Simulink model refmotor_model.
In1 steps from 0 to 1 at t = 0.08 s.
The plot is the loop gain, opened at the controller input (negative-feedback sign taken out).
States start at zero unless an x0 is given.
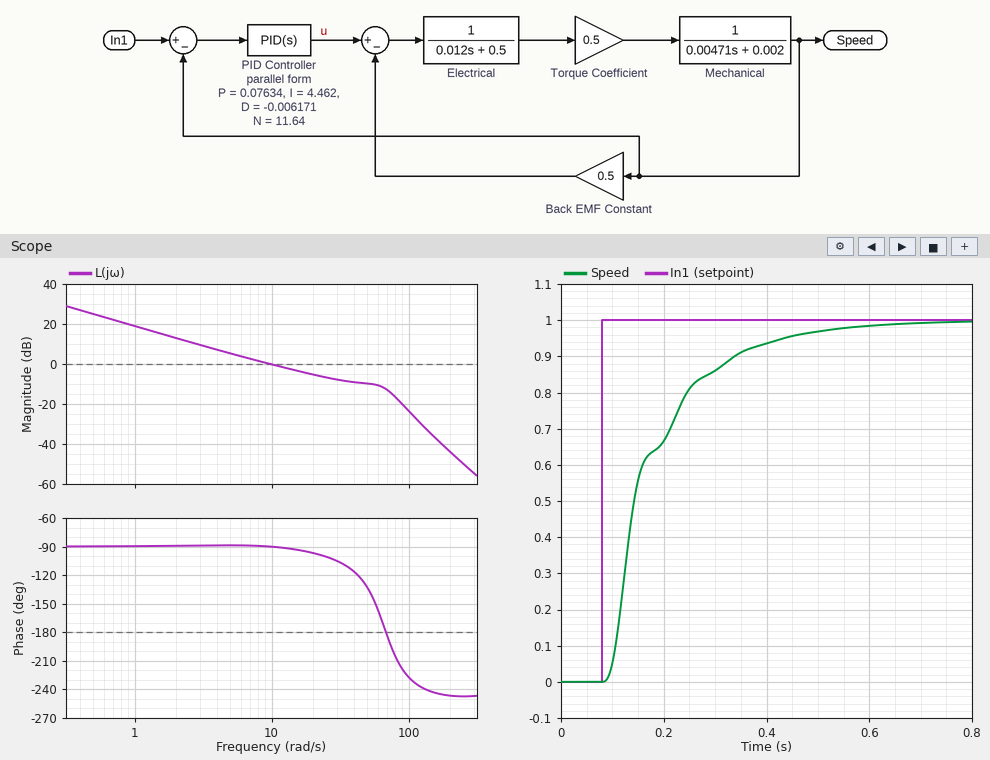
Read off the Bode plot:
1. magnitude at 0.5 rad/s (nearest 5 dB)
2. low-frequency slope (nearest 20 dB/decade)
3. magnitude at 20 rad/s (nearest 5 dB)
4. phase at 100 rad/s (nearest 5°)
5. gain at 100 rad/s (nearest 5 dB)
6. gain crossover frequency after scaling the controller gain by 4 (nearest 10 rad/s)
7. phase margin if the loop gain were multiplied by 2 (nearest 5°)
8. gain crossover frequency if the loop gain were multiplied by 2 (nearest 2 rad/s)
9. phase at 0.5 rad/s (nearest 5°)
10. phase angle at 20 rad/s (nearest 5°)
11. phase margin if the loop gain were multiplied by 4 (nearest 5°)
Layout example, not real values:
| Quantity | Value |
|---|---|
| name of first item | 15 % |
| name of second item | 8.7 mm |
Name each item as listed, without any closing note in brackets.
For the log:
| Quantity | Value |
|---|---|
| magnitude at 0.5 rad/s | 25 dB |
| low-frequency slope | -20 dB/decade |
| magnitude at 20 rad/s | -5 dB |
| phase at 100 rad/s | -225° |
| gain at 100 rad/s | -25 dB |
| gain crossover frequency after scaling the controller gain by 4 | 70 rad/s |
| phase margin if the loop gain were multiplied by 2 | 80° |
| gain crossover frequency if the loop gain were multiplied by 2 | 22 rad/s |
| phase at 0.5 rad/s | -90° |
| phase angle at 20 rad/s | -95° |
| phase margin if the loop gain were multiplied by 4 | 5° |
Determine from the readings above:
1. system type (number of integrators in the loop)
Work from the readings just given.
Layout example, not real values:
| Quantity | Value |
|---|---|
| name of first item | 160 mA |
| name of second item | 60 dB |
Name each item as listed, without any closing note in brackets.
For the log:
| Quantity | Value |
|---|---|
| system type | 1 |
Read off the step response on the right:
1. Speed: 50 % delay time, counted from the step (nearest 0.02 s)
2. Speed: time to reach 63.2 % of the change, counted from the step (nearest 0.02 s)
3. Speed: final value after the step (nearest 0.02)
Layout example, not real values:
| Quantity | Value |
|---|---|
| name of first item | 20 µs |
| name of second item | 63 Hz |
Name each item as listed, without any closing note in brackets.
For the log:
| Quantity | Value |
|---|---|
| Speed: 50 % delay time, counted from the step | 0.06 s |
| Speed: time to reach 63.2 % of the change, counted from the step | 0.10 s |
| Speed: final value after the step | 1.00 |
